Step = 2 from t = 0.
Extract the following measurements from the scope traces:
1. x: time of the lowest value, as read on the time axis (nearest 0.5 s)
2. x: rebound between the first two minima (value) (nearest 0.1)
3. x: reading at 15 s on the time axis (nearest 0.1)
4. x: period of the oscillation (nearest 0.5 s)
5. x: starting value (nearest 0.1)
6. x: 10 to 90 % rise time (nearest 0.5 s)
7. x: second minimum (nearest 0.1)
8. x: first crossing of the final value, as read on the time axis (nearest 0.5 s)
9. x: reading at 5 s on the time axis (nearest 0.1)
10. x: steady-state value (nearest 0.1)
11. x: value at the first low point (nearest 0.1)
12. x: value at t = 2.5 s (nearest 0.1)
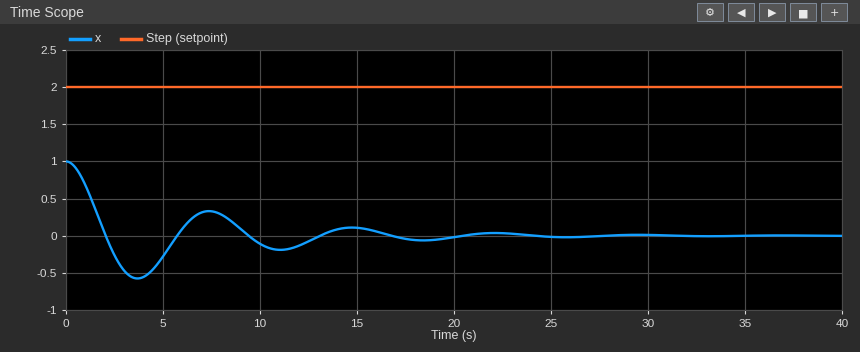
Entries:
3.5 s
0.3
0.1
7.5 s
1.0
1.5 s
-0.2
2.0 s
-0.3
0.0
-0.6
-0.3
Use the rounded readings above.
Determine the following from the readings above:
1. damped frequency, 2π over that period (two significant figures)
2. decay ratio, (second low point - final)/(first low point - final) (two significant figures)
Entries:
0.84 rad/s
0.33
